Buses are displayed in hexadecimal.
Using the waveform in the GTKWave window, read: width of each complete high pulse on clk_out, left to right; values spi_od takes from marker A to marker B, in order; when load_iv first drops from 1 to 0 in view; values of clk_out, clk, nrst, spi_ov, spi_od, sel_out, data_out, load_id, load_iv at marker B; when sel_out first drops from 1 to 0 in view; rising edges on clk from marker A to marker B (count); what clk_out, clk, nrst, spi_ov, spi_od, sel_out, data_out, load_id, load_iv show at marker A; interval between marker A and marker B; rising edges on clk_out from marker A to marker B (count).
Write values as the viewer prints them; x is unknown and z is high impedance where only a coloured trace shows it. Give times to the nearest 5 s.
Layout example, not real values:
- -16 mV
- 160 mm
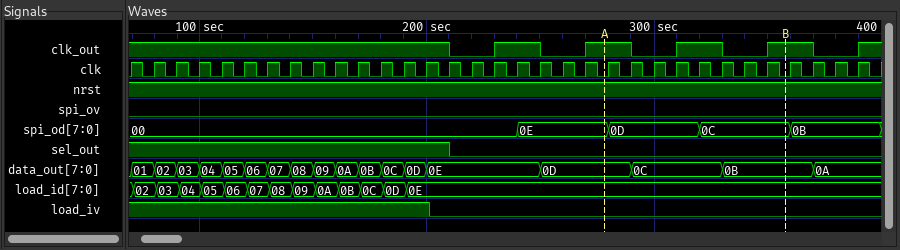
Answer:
- 20 s, 20 s, 20 s, 20 s
- 0E, 0D, 0C
- 200 s
- clk_out=1, clk=0, nrst=1, spi_ov=0, spi_od=0C, sel_out=0, data_out=0B, load_id=0E, load_iv=0
- 210 s
- 8
- clk_out=1, clk=0, nrst=1, spi_ov=0, spi_od=0E, sel_out=0, data_out=0D, load_id=0E, load_iv=0
- 80 s
- 2
